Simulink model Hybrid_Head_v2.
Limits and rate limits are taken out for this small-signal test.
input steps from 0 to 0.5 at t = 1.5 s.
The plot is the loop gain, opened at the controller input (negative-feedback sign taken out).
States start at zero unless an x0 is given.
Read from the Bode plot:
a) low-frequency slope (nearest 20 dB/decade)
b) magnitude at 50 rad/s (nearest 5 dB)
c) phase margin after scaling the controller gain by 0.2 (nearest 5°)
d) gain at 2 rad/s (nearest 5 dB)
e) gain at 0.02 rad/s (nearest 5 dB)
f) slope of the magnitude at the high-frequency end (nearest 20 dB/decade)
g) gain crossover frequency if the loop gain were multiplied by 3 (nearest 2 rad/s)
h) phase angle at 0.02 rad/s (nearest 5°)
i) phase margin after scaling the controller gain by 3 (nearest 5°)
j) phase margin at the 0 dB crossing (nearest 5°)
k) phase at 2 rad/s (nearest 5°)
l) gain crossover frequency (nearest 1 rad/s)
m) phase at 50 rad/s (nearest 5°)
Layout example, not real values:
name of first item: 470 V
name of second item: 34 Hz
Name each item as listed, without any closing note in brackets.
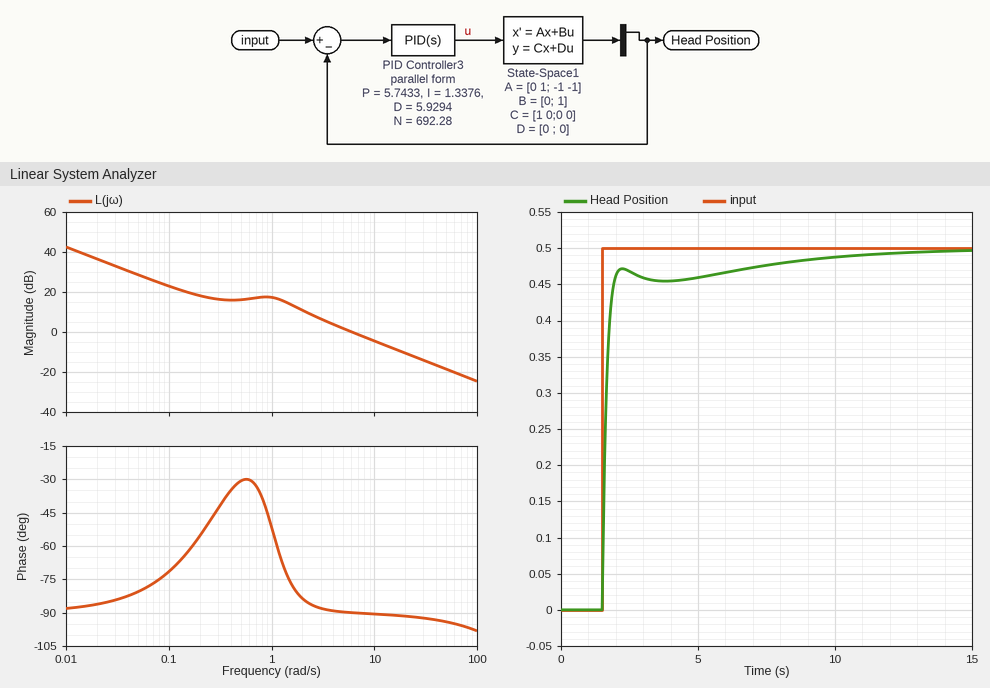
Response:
low-frequency slope: -20 dB/decade
magnitude at 50 rad/s: -20 dB
phase margin after scaling the controller gain by 0.2: 105°
gain at 2 rad/s: 10 dB
gain at 0.02 rad/s: 35 dB
slope of the magnitude at the high-frequency end: -20 dB/decade
gain crossover frequency if the loop gain were multiplied by 3: 18 rad/s
phase angle at 0.02 rad/s: -85°
phase margin after scaling the controller gain by 3: 90°
phase margin at the 0 dB crossing: 90°
phase at 2 rad/s: -85°
gain crossover frequency: 6 rad/s
phase at 50 rad/s: -95°
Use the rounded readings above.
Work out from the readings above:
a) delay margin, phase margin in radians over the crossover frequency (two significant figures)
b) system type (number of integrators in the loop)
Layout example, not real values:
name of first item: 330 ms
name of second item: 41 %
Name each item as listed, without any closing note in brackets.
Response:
delay margin, phase margin in radians over the crossover frequency: 0.26 s
system type: 1
